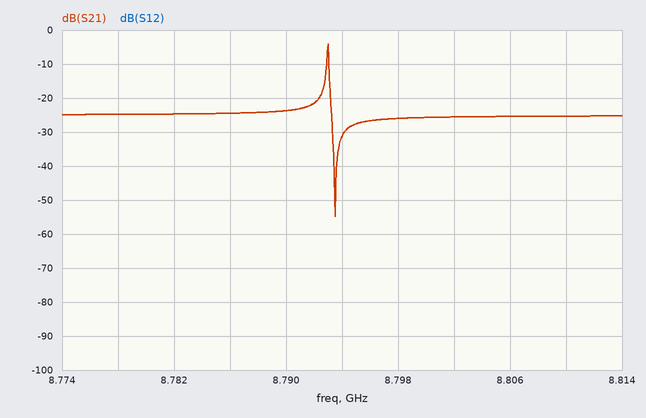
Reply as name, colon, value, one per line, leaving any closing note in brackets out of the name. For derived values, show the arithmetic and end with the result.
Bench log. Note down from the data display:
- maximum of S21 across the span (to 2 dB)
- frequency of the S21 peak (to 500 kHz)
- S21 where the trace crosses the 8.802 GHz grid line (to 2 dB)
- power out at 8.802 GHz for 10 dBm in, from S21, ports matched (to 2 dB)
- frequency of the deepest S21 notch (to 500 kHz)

maximum of S21 across the span: -4 dB
frequency of the S21 peak: 8.7930 GHz
S21 where the trace crosses the 8.802 GHz grid line: -26 dB
power out at 8.802 GHz for 10 dBm in, from S21, ports matched: 10 dBm + (-26 dB) = -16 dBm
frequency of the deepest S21 notch: 8.7935 GHz
